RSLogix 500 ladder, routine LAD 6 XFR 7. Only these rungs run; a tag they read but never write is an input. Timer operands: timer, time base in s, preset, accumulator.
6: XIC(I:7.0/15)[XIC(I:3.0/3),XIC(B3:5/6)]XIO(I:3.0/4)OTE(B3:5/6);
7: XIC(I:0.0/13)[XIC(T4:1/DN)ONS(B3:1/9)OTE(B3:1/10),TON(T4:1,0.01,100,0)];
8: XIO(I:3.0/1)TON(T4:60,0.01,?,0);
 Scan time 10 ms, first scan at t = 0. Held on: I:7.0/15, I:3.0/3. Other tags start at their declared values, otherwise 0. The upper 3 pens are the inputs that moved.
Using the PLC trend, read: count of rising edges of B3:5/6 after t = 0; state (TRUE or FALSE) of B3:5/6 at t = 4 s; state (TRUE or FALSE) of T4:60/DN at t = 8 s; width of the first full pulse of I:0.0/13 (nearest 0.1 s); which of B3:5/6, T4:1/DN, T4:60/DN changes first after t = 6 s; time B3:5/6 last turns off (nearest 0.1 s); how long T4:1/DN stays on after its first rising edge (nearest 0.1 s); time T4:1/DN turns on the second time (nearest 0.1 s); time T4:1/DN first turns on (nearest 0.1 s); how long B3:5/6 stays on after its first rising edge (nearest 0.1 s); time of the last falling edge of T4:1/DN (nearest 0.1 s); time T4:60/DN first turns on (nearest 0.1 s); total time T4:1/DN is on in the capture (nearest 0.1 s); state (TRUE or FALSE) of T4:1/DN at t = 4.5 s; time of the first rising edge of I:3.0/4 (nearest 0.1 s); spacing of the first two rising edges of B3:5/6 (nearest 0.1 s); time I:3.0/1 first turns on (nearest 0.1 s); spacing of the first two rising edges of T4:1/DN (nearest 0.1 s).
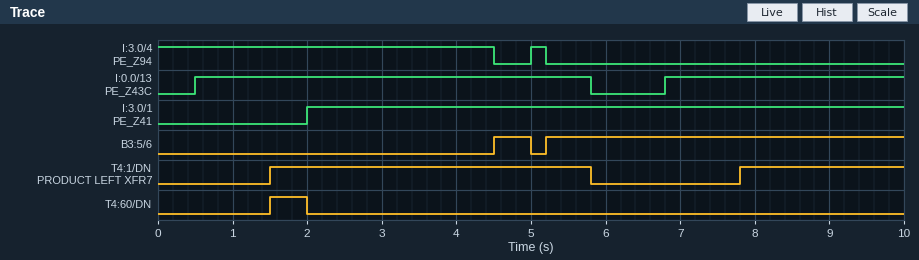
2
FALSE
FALSE
5.3 s
T4:1/DN
5.0 s
4.3 s
7.8 s
1.5 s
0.5 s
5.8 s
1.5 s
6.5 s
TRUE
5.0 s
0.7 s
2.0 s
6.3 s
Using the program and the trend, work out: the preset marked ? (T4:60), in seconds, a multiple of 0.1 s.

1.5 s
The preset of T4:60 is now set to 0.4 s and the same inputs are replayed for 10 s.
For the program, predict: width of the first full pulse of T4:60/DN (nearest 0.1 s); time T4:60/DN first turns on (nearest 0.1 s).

1.6 s
0.4 s
